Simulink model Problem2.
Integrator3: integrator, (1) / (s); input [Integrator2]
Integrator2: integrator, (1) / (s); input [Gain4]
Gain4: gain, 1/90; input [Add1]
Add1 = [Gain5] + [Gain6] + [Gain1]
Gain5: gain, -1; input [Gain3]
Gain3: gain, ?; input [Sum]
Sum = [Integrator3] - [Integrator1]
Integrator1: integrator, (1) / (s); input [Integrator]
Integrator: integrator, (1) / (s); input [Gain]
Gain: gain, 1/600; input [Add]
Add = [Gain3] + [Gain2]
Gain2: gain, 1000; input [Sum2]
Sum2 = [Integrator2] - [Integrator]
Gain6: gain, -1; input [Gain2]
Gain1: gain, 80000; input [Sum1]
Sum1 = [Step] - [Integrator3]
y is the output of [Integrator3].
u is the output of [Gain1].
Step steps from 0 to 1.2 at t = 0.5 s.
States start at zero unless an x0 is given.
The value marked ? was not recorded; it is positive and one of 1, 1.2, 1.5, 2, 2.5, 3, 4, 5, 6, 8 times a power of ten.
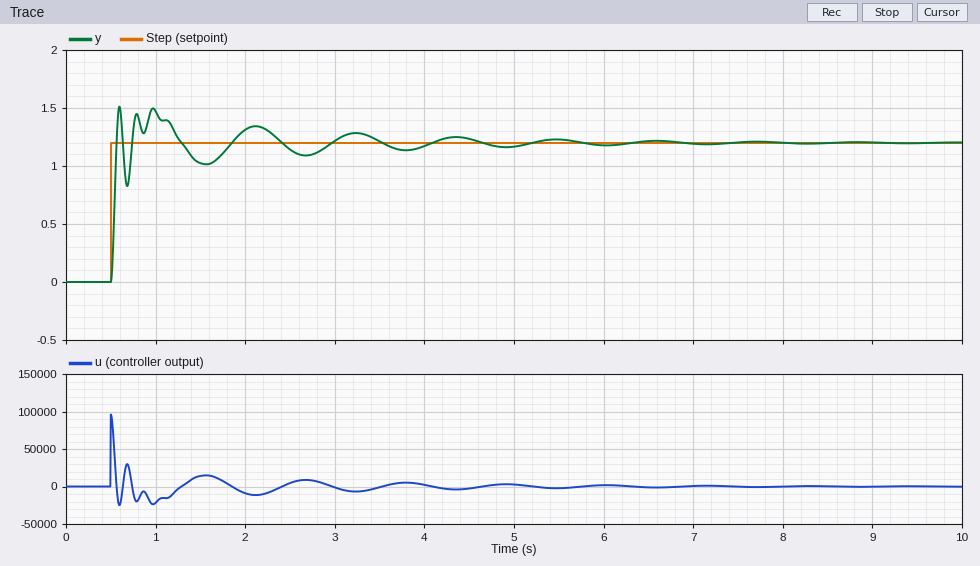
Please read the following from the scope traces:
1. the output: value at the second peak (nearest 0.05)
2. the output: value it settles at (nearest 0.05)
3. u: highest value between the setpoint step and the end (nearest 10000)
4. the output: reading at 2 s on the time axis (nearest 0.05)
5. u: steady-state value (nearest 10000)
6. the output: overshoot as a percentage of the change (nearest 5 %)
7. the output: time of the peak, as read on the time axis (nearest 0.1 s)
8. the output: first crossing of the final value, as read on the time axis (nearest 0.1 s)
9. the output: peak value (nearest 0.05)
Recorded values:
1.45
1.20
100000
1.30
0
25 %
0.6 s
0.6 s
1.50
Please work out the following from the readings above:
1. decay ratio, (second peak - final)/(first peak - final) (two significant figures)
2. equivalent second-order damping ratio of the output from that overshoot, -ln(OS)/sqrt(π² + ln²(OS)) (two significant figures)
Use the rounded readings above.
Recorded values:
0.83
0.40
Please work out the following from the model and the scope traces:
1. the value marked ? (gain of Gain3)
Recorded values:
25000
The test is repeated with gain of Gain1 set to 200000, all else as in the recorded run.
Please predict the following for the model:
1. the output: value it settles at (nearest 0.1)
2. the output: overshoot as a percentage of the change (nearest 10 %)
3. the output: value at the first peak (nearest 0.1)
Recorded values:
1.2
50 %
1.8
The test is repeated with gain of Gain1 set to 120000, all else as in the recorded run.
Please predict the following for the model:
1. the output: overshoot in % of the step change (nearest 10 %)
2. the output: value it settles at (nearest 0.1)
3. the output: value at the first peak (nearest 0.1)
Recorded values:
40 %
1.2
1.7
